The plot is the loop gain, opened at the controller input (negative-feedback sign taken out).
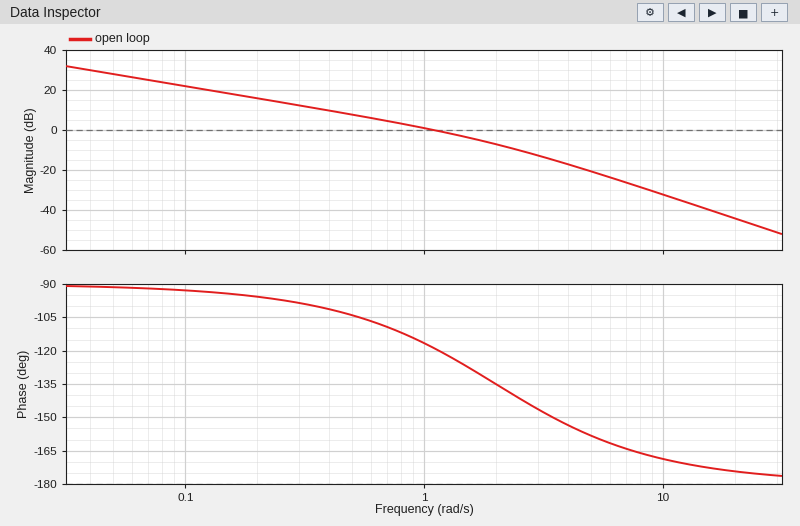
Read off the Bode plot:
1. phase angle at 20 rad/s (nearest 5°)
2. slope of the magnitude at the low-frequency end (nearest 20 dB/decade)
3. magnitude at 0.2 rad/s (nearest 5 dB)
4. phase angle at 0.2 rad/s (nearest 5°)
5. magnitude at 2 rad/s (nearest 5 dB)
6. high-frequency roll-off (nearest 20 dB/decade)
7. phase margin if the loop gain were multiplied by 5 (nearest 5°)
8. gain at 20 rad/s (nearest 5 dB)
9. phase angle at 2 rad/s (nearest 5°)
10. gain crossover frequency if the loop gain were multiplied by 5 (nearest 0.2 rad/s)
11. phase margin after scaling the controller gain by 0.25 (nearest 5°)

-175°
-20 dB/decade
15 dB
-95°
-5 dB
-40 dB/decade
30°
-45 dB
-135°
3.2 rad/s
80°
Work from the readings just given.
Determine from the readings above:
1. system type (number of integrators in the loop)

1
